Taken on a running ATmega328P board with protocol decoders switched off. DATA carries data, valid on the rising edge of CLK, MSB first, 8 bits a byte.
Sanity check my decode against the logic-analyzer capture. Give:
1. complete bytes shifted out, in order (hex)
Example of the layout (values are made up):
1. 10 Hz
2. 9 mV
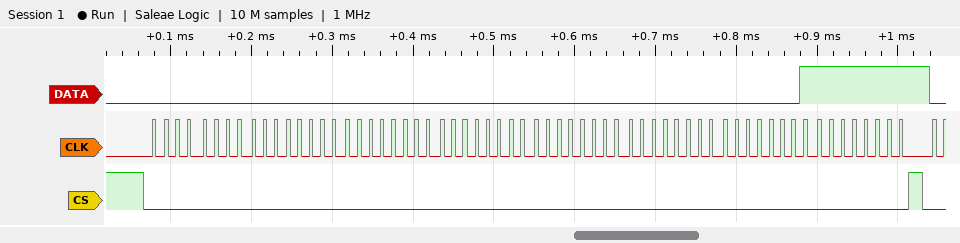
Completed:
1. 00 00 00 00 00 00 01 FF
